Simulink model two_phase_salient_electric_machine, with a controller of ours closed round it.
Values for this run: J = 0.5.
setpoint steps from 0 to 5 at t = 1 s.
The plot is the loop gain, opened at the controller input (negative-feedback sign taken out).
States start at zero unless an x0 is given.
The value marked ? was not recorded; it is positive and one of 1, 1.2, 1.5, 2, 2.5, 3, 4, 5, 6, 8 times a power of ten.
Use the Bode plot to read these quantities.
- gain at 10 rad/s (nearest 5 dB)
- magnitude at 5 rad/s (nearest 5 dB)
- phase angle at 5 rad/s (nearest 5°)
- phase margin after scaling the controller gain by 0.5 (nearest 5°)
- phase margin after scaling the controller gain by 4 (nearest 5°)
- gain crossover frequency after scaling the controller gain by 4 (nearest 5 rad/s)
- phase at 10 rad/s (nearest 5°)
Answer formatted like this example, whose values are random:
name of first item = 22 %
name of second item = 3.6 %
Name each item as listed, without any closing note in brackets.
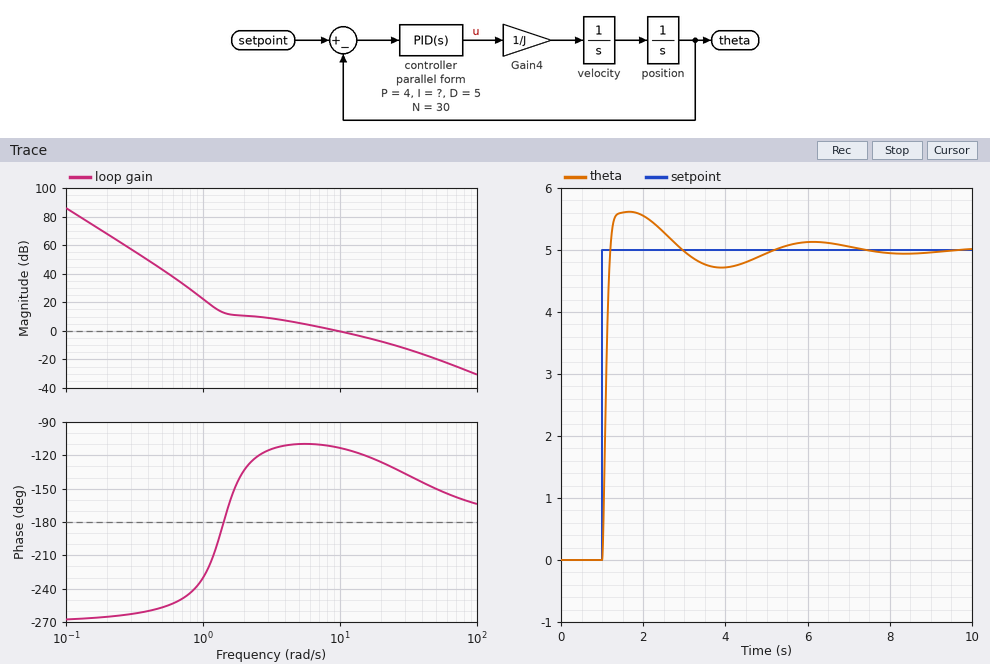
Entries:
gain at 10 rad/s = 0 dB
magnitude at 5 rad/s = 5 dB
phase angle at 5 rad/s = -110°
phase margin after scaling the controller gain by 0.5 = 70°
phase margin after scaling the controller gain by 4 = 45°
gain crossover frequency after scaling the controller gain by 4 = 30 rad/s
phase at 10 rad/s = -115°
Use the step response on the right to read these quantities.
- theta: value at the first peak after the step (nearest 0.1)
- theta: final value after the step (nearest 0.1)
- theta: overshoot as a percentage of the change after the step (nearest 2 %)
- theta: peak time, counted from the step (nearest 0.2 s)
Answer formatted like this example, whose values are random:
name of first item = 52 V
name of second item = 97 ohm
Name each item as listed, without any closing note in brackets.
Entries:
theta: value at the first peak after the step = 5.6
theta: final value after the step = 5.0
theta: overshoot as a percentage of the change after the step = 12 %
theta: peak time, counted from the step = 0.6 s
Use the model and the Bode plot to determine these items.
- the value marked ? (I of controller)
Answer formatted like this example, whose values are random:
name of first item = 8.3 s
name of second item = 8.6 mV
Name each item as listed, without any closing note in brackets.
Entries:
the value marked ? = 10
